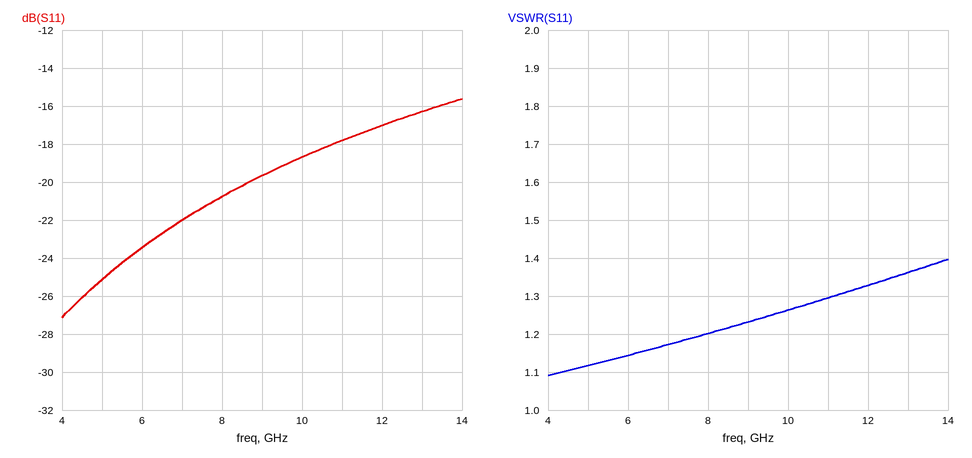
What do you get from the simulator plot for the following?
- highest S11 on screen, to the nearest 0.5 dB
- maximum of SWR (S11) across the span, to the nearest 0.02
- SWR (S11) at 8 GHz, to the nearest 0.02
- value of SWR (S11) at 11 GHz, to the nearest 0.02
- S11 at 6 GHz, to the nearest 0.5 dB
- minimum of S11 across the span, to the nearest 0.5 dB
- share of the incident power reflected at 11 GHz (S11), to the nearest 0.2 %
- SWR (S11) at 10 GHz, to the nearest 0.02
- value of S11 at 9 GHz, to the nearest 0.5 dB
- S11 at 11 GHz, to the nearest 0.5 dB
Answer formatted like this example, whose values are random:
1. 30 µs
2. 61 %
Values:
1. -15.5 dB
2. 1.40
3. 1.20
4. 1.30
5. -23.5 dB
6. -27.0 dB
7. 1.6 %
8. 1.26
9. -19.5 dB
10. -18.0 dB
